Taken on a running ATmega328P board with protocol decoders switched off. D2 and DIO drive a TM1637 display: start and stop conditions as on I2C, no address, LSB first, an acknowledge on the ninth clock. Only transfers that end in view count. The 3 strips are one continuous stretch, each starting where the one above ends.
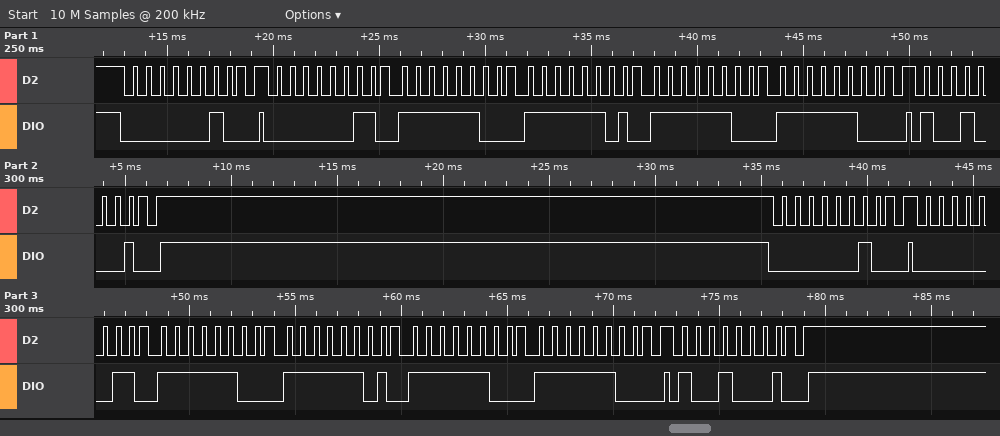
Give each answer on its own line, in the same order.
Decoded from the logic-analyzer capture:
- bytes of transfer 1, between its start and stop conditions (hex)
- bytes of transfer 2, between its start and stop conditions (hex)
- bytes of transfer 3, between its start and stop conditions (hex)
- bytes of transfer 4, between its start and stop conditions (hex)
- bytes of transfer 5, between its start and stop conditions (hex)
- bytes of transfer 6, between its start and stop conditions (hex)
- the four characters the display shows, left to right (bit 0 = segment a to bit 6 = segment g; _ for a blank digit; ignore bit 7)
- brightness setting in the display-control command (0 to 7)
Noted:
40
C0 3F BF 3F 3F
89
40
C0 3F BF 3F 3F
89
0000
1
